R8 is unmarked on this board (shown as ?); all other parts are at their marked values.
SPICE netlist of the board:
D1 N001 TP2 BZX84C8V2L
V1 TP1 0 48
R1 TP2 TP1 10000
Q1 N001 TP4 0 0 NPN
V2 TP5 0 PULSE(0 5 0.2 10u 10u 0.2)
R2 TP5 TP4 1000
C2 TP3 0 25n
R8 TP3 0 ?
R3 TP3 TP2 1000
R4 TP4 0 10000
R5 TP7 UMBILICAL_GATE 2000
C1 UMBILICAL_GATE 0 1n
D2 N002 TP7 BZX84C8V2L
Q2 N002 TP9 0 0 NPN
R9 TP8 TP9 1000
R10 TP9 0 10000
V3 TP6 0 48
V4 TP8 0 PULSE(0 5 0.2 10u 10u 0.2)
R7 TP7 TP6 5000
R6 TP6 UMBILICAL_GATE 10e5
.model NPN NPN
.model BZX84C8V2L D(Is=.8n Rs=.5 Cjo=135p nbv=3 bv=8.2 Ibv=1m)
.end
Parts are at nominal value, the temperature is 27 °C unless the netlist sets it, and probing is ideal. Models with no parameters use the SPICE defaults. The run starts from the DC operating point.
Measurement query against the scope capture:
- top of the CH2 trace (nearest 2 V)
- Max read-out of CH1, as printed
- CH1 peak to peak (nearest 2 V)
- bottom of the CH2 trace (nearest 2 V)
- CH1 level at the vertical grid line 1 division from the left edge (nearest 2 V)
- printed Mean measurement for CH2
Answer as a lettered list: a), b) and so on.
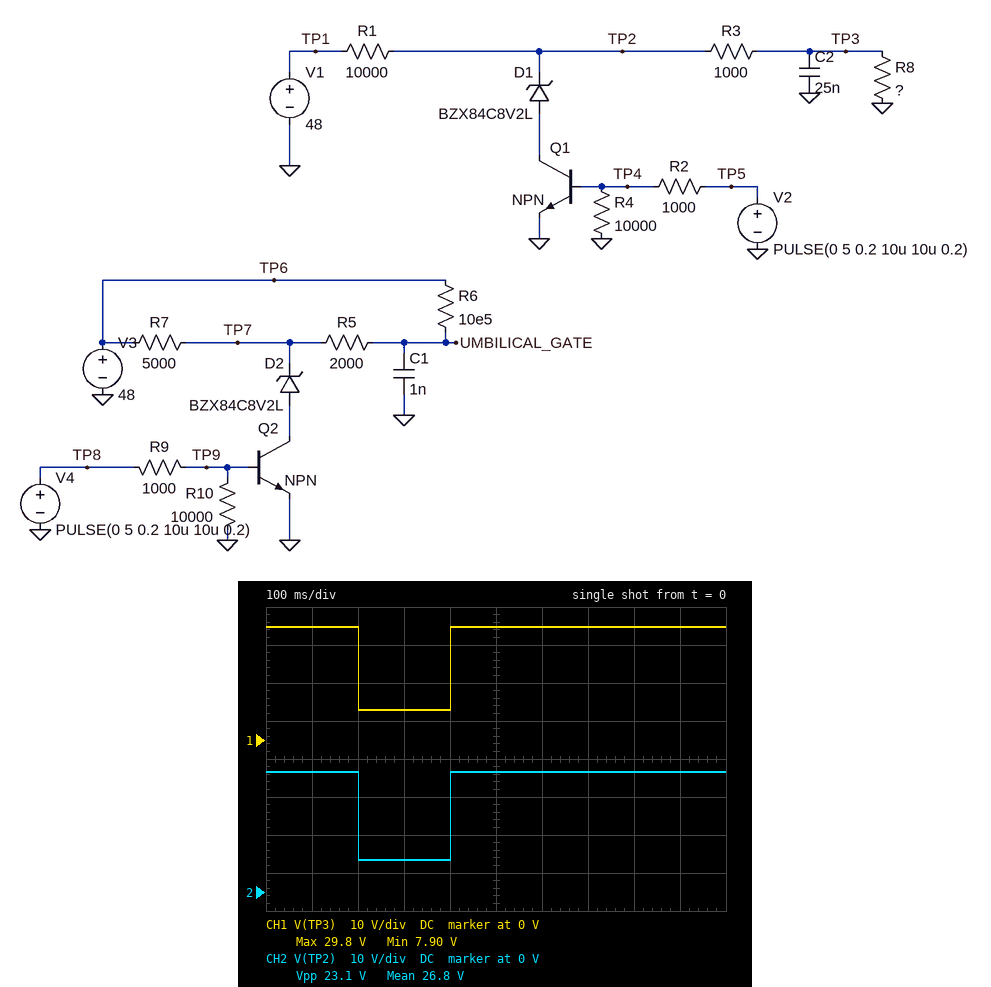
a) 32 V
b) 29.8 V
c) 22 V
d) 8 V
e) 30 V
f) 26.8 V
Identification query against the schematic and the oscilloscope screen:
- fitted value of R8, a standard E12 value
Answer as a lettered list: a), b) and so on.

a) 18 kΩ
